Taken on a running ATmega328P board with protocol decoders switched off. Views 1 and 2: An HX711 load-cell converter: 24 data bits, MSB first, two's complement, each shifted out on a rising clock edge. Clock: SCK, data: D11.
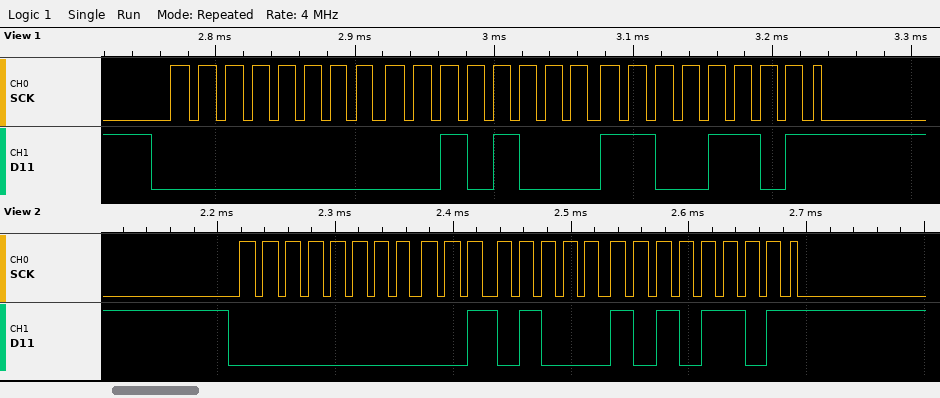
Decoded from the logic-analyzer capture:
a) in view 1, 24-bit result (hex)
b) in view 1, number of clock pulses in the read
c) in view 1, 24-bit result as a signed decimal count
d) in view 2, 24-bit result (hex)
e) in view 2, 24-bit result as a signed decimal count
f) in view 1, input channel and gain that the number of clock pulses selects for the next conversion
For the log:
0x0028CD
25
10445
0x0028AD
10413
channel A, gain 128
